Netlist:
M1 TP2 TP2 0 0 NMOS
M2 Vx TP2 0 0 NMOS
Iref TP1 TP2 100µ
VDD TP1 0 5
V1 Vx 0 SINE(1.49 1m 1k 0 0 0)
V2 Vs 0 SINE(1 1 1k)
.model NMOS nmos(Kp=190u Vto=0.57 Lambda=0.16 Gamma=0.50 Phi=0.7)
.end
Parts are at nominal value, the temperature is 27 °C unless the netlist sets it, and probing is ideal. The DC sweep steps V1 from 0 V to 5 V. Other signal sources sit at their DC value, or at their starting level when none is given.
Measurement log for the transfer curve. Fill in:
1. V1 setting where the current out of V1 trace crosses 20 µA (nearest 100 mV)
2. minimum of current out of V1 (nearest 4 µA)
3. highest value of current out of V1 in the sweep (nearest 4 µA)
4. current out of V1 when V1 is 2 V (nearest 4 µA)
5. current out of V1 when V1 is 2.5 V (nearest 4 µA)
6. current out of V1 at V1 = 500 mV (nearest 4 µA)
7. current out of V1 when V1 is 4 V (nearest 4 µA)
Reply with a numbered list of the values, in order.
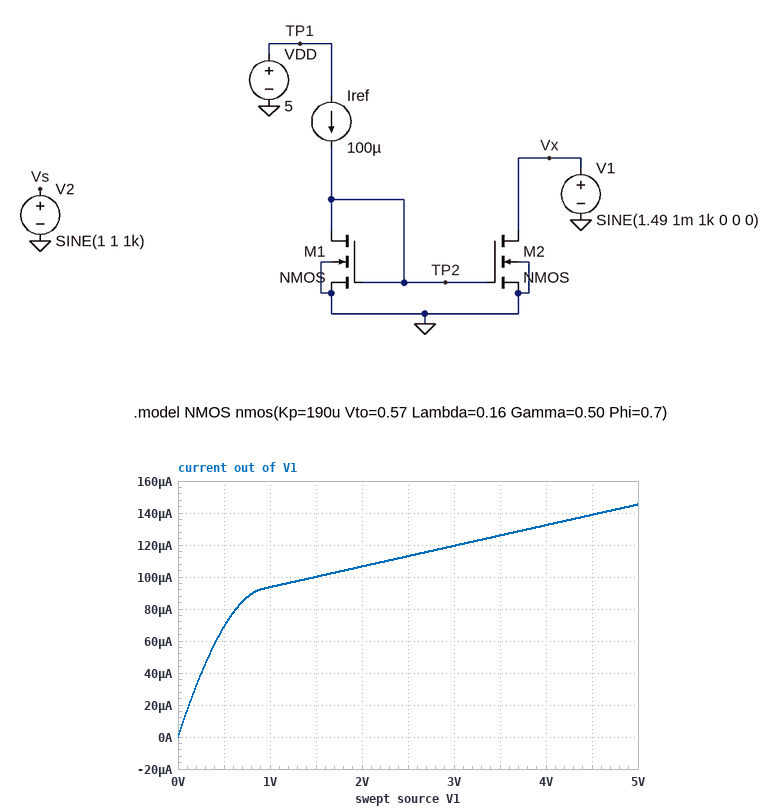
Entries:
1. 100 mV
2. 0 A
3. 144 µA
4. 108 µA
5. 112 µA
6. 68 µA
7. 132 µA
